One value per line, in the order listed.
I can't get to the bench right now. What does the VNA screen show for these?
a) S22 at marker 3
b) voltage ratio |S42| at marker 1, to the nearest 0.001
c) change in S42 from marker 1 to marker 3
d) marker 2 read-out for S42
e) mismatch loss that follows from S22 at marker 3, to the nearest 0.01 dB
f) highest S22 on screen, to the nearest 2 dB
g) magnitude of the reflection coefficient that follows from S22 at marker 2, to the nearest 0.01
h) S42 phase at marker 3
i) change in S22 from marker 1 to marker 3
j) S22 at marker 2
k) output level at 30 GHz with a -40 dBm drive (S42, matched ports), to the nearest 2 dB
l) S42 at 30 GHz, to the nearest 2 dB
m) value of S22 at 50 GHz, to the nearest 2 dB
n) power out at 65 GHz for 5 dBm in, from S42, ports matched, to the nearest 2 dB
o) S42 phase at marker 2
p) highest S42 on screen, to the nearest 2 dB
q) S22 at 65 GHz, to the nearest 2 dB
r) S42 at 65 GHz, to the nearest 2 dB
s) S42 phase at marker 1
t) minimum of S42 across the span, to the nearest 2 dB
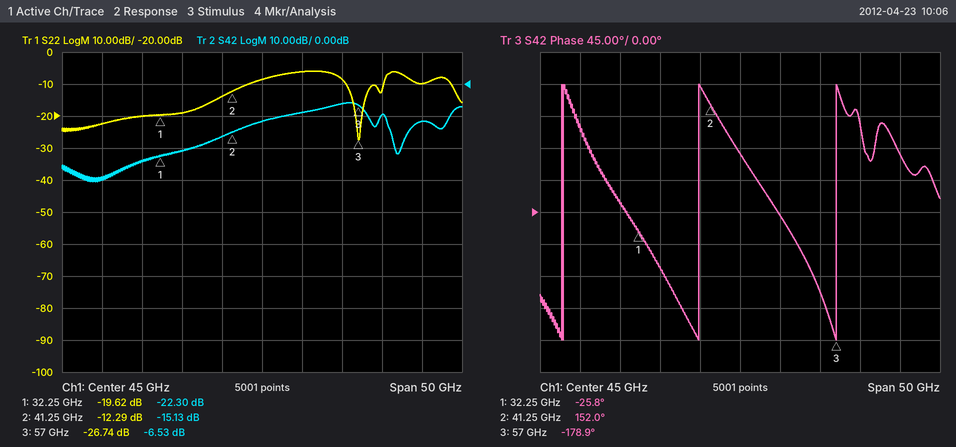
-26.74 dB
0.077
15.77 dB
-15.13 dB
0.01 dB
-6 dB
0.24
-178.9°
-7.12 dB
-12.29 dB
-64 dBm
-24 dB
-6 dB
-6 dBm
152.0°
-6 dB
-10 dB
-12 dB
-25.8°
-30 dB
